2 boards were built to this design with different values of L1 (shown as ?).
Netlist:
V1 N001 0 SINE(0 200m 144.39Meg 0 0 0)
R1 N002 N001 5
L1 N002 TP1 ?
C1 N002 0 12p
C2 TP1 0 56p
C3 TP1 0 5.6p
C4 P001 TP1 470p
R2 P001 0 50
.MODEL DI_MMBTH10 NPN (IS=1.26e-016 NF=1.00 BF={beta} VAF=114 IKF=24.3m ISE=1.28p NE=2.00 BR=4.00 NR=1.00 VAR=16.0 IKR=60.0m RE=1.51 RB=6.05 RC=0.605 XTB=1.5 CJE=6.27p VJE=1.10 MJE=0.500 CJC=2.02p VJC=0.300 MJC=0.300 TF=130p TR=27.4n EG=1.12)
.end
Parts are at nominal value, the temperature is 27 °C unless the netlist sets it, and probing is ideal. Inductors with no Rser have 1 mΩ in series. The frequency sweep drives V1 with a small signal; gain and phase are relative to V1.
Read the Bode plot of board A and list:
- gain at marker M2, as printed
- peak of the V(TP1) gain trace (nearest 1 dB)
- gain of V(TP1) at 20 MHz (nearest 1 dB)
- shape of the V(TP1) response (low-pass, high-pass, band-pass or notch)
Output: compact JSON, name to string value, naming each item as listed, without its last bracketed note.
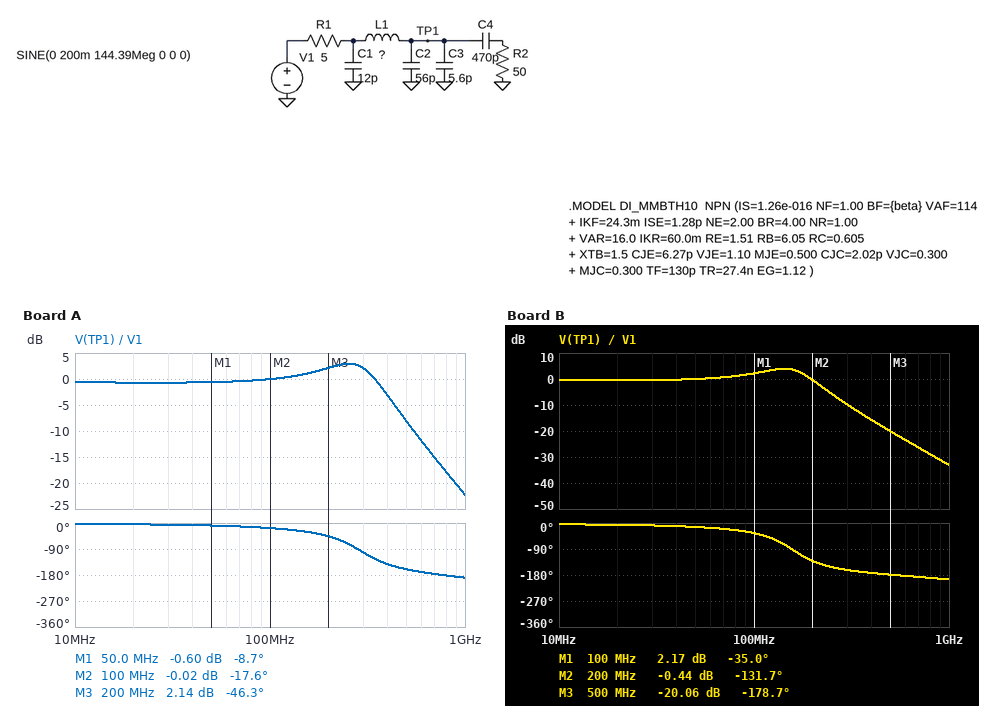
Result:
{"gain at marker M2, as printed": "-0.02 dB", "peak of the V(TP1) gain trace": "3 dB", "gain of V(TP1) at 20 MHz": "-1 dB", "shape of the V(TP1) response": "low-pass"}
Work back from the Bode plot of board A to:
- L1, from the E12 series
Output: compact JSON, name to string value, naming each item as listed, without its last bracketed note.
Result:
{"L1, from the E12 series": "5.6 nH"}
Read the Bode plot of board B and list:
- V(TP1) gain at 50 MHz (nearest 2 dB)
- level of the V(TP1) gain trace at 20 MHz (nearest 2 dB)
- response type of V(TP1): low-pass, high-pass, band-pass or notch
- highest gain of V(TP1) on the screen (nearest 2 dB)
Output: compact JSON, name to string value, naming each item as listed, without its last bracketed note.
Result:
{"V(TP1) gain at 50 MHz": "0 dB", "level of the V(TP1) gain trace at 20 MHz": "0 dB", "response type of V(TP1): low-pass, high-pass, band-pass or notch": "low-pass", "highest gain of V(TP1) on the screen": "4 dB"}
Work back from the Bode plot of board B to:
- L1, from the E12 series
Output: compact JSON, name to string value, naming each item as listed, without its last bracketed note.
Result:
{"L1, from the E12 series": "18 nH"}
